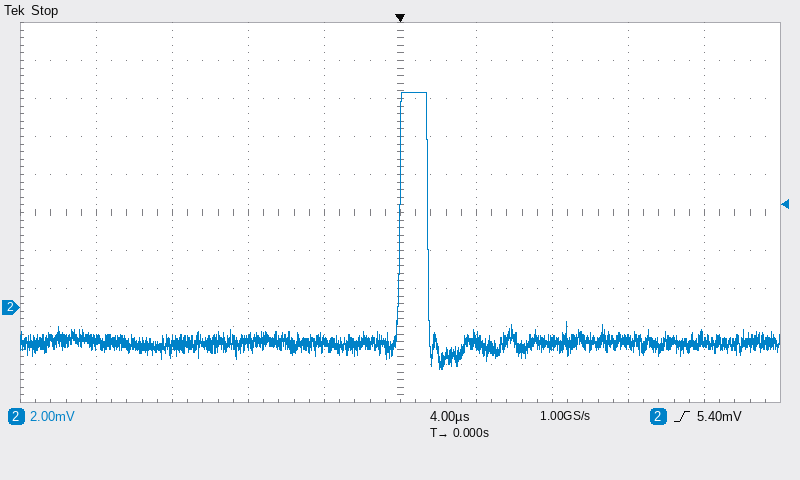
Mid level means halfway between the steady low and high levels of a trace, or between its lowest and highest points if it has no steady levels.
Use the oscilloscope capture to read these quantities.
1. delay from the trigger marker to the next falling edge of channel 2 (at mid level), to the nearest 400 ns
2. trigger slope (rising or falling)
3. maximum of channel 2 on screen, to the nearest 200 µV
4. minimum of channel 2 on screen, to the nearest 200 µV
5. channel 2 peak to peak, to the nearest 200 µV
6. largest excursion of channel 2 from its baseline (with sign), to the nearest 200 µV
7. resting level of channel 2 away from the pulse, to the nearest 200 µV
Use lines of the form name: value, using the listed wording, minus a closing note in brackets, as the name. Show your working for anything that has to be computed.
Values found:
delay from the trigger marker to the next falling edge of channel 2 (at mid level), to the nearest 400 ns: 1.6 µs
trigger slope: rising
maximum of channel 2 on screen, to the nearest 200 µV: 11.4 mV
minimum of channel 2 on screen, to the nearest 200 µV: -3.2 mV
channel 2 peak to peak, to the nearest 200 µV: 11.4 mV − (-3.2 mV) = 14.6 mV
largest excursion of channel 2 from its baseline (with sign), to the nearest 200 µV: 11.4 mV − (-1.8 mV) = +13.2 mV
resting level of channel 2 away from the pulse, to the nearest 200 µV: -1.8 mV
